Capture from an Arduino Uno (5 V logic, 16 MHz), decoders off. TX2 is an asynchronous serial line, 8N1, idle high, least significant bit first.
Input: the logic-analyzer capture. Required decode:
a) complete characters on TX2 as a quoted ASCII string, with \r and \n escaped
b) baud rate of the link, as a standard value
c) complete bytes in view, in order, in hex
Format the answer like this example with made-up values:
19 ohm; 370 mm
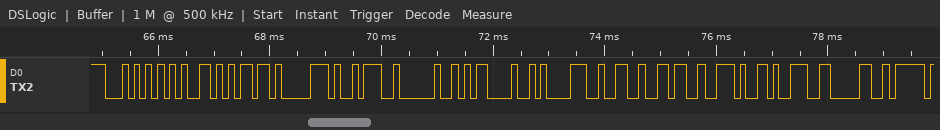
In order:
"Temp: \r\n26.90"; 9600 baud; 0x54 0x65 0x6D 0x70 0x3A 0x20 0x0D 0x0A 0x32 0x36 0x2E 0x39 0x30
